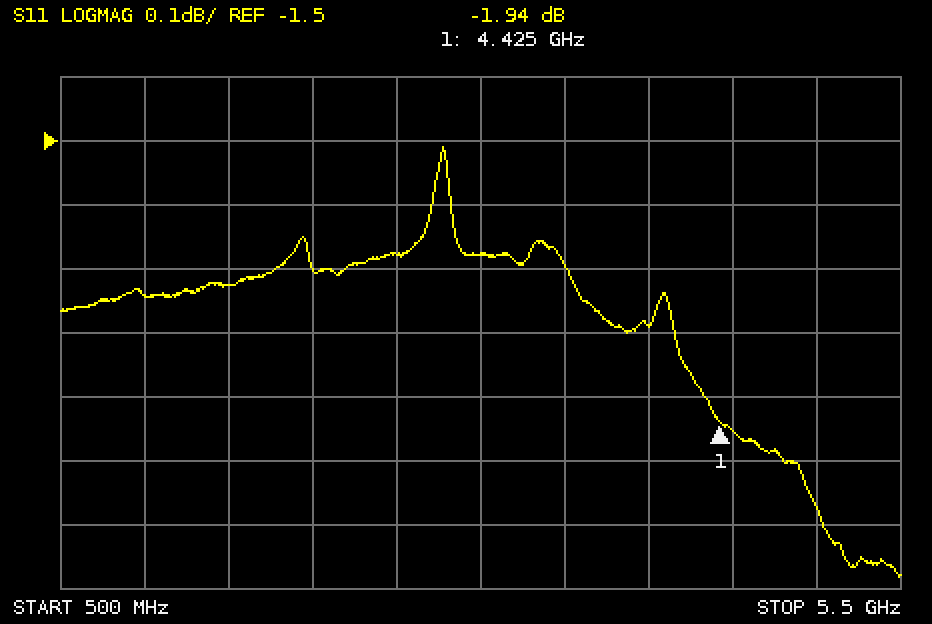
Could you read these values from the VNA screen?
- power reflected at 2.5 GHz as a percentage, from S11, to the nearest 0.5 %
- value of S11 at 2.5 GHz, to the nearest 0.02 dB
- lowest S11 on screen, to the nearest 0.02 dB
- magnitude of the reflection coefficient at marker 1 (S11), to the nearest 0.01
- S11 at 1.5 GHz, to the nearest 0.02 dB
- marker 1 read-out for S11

68.0 %
-1.68 dB
-2.18 dB
0.80
-1.72 dB
-1.94 dB
